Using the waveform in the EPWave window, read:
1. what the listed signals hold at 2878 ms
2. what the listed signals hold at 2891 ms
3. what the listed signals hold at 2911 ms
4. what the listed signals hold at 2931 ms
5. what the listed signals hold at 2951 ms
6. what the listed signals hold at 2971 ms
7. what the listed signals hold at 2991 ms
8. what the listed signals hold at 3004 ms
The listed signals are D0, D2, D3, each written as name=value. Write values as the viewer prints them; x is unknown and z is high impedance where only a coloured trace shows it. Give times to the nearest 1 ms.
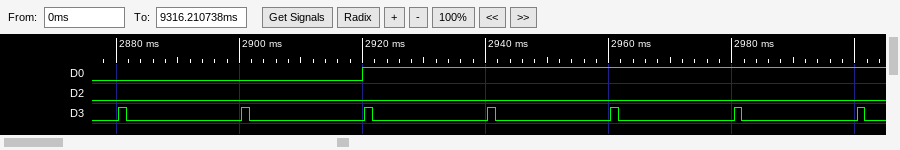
D0=0, D2=0, D3=0
D0=0, D2=0, D3=0
D0=0, D2=0, D3=0
D0=1, D2=0, D3=0
D0=1, D2=0, D3=0
D0=1, D2=0, D3=0
D0=1, D2=0, D3=0
D0=1, D2=0, D3=0
